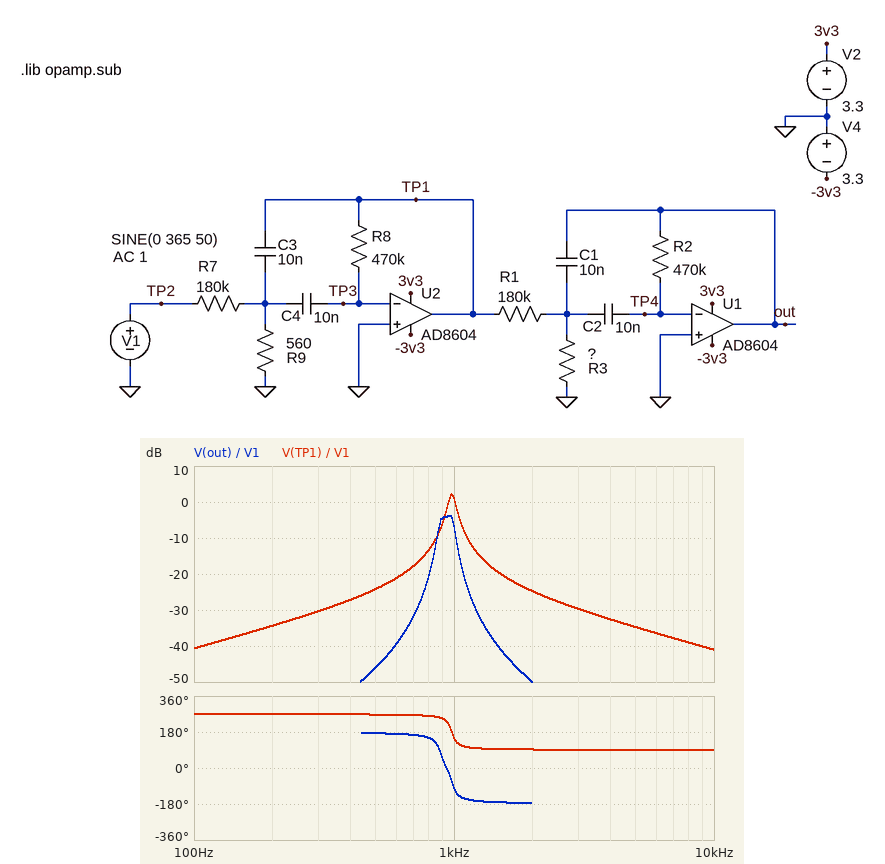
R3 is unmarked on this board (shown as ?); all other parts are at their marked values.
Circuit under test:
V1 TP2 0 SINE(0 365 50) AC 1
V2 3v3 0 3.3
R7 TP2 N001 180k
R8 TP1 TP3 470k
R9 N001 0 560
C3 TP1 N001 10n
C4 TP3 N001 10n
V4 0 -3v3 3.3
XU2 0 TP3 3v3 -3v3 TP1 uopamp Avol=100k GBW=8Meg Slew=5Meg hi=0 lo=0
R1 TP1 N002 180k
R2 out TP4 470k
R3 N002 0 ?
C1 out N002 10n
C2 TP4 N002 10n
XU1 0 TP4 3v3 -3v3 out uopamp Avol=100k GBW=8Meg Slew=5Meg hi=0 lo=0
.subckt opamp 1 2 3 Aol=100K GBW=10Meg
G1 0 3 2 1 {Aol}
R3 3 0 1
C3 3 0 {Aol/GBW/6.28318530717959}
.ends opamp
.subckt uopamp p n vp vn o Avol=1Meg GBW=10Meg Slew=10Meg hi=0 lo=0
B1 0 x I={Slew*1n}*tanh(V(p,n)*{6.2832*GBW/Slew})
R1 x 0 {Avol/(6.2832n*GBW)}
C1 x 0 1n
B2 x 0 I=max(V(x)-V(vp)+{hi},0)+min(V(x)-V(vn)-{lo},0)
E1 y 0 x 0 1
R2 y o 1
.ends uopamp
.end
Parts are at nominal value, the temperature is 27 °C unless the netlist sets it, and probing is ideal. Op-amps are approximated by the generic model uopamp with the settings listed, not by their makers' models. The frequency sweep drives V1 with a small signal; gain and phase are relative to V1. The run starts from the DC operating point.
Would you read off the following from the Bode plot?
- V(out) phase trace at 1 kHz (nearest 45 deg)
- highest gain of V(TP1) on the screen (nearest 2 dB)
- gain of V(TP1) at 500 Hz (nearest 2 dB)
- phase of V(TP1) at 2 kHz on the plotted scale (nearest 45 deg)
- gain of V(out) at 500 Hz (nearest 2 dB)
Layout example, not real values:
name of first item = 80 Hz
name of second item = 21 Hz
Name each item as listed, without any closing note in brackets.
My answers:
V(out) phase trace at 1 kHz = -90 deg
highest gain of V(TP1) on the screen = 2 dB
gain of V(TP1) at 500 Hz = -24 dB
phase of V(TP1) at 2 kHz on the plotted scale = 90 deg
gain of V(out) at 500 Hz = -46 dB
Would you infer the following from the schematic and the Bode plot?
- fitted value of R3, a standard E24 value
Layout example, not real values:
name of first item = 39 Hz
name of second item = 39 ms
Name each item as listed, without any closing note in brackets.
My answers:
fitted value of R3, a standard E24 value = 680 Ω
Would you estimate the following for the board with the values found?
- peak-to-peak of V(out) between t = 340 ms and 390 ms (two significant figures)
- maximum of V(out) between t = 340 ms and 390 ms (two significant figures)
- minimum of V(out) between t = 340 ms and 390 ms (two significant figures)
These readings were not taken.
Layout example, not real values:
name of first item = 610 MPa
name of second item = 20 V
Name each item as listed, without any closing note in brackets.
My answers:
peak-to-peak of V(out) between t = 340 ms and 390 ms = 19 mV
maximum of V(out) between t = 340 ms and 390 ms = 9.3 mV
minimum of V(out) between t = 340 ms and 390 ms = -9.3 mV
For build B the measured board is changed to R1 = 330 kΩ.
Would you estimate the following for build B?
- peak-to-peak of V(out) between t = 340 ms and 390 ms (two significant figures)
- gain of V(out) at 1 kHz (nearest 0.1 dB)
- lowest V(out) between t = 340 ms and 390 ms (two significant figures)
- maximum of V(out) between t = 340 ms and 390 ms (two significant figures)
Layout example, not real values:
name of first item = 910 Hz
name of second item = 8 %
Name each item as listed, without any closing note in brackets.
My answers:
peak-to-peak of V(out) between t = 340 ms and 390 ms = 10 mV
gain of V(out) at 1 kHz = -12.1 dB
lowest V(out) between t = 340 ms and 390 ms = -5.1 mV
maximum of V(out) between t = 340 ms and 390 ms = 5.1 mV
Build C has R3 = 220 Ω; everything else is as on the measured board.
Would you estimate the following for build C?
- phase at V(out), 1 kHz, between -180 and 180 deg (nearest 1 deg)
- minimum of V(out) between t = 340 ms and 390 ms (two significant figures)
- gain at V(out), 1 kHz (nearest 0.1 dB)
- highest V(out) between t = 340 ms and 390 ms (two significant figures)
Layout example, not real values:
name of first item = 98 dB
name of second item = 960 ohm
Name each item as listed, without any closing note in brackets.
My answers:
phase at V(out), 1 kHz, between -180 and 180 deg = 58 deg
minimum of V(out) between t = 340 ms and 390 ms = -3.0 mV
gain at V(out), 1 kHz = -23.2 dB
highest V(out) between t = 340 ms and 390 ms = 3.0 mV
